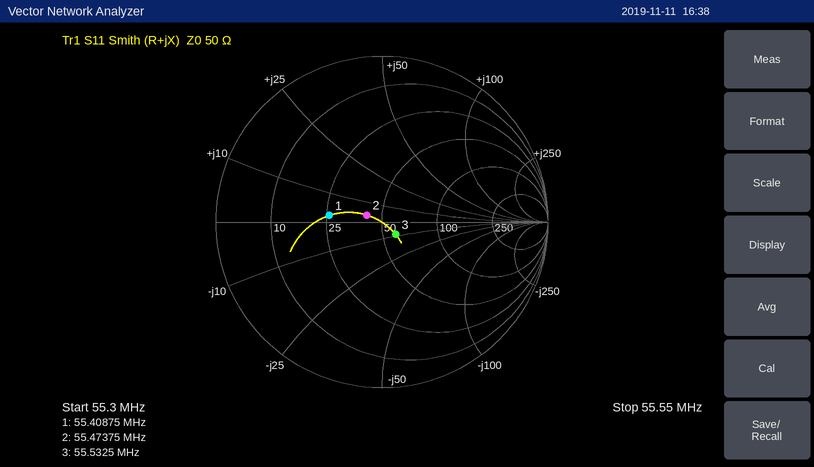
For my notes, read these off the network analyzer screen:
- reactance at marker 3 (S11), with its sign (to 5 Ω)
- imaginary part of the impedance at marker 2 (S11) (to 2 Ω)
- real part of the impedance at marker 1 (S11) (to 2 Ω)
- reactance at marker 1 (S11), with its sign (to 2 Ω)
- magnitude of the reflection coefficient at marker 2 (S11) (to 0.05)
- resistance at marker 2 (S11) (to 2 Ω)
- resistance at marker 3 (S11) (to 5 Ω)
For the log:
-10 Ω
+4 Ω
26 Ω
+2 Ω
0.10
42 Ω
60 Ω
